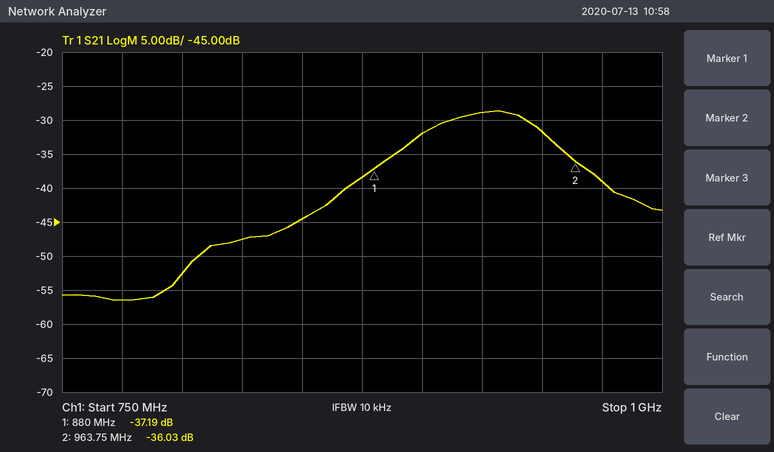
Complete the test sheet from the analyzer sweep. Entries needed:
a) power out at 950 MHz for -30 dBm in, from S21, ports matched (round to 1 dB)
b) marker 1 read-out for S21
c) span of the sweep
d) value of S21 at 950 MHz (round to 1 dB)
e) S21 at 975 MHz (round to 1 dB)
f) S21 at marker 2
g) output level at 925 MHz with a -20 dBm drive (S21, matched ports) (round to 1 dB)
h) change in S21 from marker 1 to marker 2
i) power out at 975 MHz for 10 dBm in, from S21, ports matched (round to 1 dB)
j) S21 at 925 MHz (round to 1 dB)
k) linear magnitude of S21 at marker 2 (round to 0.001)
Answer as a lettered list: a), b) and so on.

a) -62 dBm
b) -37.19 dB
c) 250 MHz
d) -32 dB
e) -39 dB
f) -36.03 dB
g) -49 dBm
h) 1.16 dB
i) -29 dBm
j) -29 dB
k) 0.016
